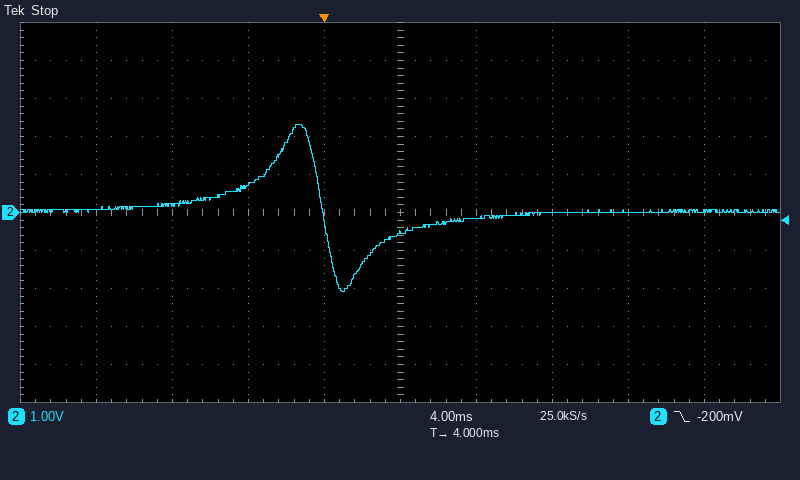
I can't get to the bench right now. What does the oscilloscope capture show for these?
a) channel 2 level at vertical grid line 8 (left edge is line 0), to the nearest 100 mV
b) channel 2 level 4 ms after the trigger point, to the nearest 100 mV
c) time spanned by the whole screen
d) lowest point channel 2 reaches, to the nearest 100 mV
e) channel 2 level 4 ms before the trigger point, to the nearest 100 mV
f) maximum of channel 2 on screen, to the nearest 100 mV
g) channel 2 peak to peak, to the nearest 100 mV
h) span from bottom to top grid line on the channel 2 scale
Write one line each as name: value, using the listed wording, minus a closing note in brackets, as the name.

channel 2 level at vertical grid line 8 (left edge is line 0), to the nearest 100 mV: 0.0 V
channel 2 level 4 ms after the trigger point, to the nearest 100 mV: -600 mV
time spanned by the whole screen: 40 ms
lowest point channel 2 reaches, to the nearest 100 mV: -2.1 V
channel 2 level 4 ms before the trigger point, to the nearest 100 mV: 700 mV
maximum of channel 2 on screen, to the nearest 100 mV: 2.3 V
channel 2 peak to peak, to the nearest 100 mV: 4.4 V
span from bottom to top grid line on the channel 2 scale: 10 V
